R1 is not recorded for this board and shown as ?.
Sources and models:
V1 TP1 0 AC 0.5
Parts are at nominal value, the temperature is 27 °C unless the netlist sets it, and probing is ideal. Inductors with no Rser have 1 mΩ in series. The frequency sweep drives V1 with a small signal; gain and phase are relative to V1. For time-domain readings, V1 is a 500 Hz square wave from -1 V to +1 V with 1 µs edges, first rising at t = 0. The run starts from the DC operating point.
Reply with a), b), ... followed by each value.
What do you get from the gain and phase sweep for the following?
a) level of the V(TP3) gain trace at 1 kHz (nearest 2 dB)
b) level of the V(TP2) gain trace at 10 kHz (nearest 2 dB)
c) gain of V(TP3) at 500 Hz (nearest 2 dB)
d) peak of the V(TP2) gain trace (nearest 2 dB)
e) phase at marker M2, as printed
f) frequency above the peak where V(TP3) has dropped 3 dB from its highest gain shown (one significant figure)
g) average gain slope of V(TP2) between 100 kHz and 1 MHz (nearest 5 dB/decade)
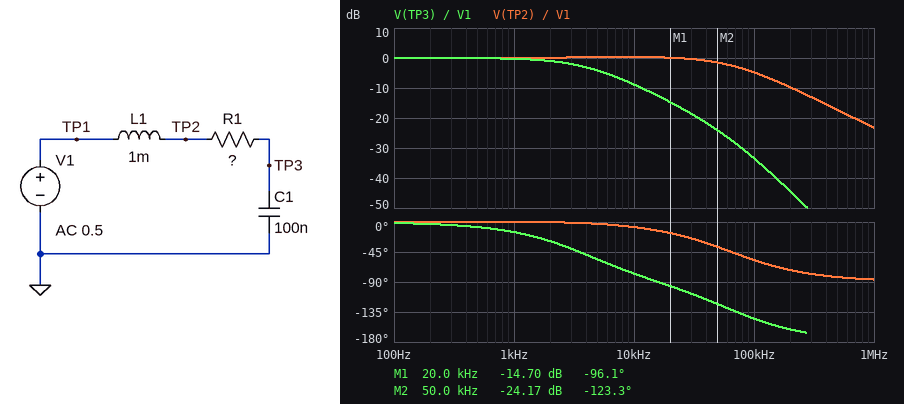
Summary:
a) 0 dB
b) 0 dB
c) 0 dB
d) 0 dB
e) -123.3 deg
f) 4 kHz
g) -20 dB/decade
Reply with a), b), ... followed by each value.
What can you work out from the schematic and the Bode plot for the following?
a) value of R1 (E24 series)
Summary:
a) 430 Ω
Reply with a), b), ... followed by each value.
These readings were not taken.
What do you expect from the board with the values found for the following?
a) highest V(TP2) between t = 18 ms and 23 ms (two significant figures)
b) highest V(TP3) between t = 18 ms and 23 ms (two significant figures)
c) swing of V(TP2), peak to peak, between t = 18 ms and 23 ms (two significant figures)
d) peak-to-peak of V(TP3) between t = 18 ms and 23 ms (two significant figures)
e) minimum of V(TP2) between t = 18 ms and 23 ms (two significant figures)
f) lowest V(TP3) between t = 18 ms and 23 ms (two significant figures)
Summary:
a) 1.1 V
b) 1.0 V
c) 2.2 V
d) 2.0 V
e) -1.1 V
f) -1.0 V
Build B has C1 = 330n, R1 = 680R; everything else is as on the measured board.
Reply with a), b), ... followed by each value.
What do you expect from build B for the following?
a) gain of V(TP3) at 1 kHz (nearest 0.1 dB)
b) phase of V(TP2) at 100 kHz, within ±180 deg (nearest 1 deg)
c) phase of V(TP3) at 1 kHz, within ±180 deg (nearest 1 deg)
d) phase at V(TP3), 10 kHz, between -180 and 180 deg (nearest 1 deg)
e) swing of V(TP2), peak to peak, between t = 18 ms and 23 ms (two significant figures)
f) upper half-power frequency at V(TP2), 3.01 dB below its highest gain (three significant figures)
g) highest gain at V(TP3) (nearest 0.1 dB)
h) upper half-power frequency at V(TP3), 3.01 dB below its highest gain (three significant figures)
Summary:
a) -4.7 dB
b) -43 deg
c) -55 deg
d) -91 deg
e) 2.0 V
f) 108 kHz
g) 0 dB
h) 714 Hz
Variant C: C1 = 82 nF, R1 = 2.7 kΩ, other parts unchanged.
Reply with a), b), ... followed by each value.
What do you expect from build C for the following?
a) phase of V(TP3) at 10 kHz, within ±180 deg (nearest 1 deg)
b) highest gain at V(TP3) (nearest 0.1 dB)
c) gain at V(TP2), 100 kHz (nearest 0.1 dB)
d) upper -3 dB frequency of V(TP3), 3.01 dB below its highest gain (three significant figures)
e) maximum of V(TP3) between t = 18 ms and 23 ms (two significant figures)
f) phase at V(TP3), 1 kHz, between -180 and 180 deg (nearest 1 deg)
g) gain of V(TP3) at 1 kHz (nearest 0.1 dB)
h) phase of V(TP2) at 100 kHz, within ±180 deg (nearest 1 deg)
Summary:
a) -87 deg
b) 0 dB
c) -0.2 dB
d) 720 Hz
e) 980 mV
f) -54 deg
g) -4.7 dB
h) -13 deg
